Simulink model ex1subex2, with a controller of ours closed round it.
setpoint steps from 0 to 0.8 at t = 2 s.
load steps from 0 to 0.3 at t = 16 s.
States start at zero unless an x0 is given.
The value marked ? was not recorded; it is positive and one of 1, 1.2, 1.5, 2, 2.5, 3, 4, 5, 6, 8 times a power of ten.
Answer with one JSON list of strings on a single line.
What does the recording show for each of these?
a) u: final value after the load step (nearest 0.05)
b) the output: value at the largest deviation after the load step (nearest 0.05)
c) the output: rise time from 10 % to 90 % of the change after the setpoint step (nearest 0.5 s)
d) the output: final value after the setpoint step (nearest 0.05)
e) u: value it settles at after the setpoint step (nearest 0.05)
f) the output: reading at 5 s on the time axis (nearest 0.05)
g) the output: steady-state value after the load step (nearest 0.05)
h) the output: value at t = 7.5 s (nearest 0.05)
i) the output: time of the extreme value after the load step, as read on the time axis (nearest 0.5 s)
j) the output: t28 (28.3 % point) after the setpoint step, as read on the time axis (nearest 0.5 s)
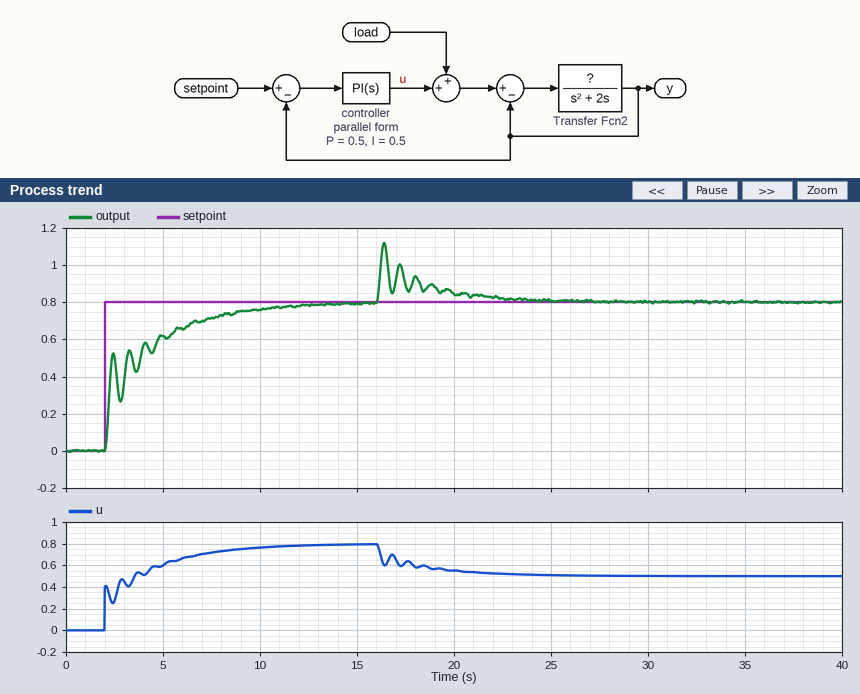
["0.50", "1.10", "5.5 s", "0.80", "0.80", "0.60", "0.80", "0.70", "16.5 s", "2.0 s"]
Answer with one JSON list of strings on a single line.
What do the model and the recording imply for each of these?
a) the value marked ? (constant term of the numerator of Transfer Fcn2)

["40"]
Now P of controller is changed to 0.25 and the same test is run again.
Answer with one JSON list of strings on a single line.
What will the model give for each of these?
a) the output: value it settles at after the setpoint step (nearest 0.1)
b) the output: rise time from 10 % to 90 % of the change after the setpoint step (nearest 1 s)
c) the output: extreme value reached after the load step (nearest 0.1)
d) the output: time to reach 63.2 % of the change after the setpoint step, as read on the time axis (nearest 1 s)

["0.8", "5 s", "1.2", "4 s"]
